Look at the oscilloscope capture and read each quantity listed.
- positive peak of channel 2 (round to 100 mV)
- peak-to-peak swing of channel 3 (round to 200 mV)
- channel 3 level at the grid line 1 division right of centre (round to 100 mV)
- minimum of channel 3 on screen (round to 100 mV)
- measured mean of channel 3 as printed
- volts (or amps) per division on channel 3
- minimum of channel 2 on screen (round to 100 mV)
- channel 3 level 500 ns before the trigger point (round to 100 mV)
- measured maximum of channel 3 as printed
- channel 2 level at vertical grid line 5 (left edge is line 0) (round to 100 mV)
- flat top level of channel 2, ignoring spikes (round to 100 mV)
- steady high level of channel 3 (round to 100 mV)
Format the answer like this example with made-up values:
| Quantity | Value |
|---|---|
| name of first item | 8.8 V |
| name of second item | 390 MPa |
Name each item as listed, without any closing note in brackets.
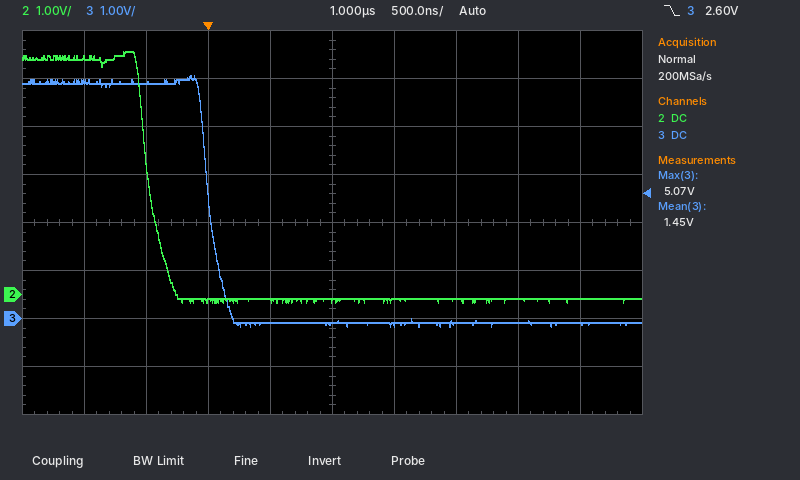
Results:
| Quantity | Value |
|---|---|
| positive peak of channel 2 | 5.1 V |
| peak-to-peak swing of channel 3 | 5.2 V |
| channel 3 level at the grid line 1 division right of centre | -100 mV |
| minimum of channel 3 on screen | -200 mV |
| measured mean of channel 3 as printed | 1.45 V |
| volts (or amps) per division on channel 3 | 1 V |
| minimum of channel 2 on screen | -200 mV |
| channel 3 level 500 ns before the trigger point | 4.9 V |
| measured maximum of channel 3 as printed | 5.07 V |
| channel 2 level at vertical grid line 5 (left edge is line 0) | -100 mV |
| flat top level of channel 2, ignoring spikes | 4.9 V |
| steady high level of channel 3 | 4.9 V |
